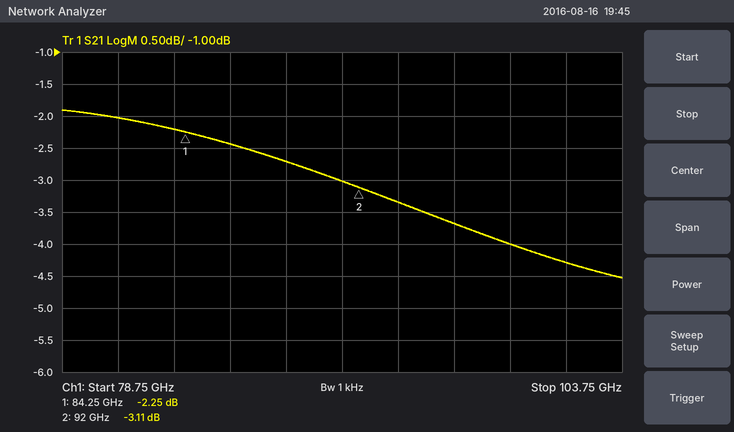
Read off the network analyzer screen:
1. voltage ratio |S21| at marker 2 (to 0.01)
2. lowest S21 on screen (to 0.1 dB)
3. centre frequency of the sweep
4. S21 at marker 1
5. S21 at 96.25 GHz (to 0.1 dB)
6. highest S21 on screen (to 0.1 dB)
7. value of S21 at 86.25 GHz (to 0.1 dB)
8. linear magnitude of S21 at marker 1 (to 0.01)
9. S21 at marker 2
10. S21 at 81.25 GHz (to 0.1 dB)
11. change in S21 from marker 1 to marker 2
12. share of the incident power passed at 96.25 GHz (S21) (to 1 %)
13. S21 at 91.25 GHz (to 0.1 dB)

0.70
-4.5 dB
91.25 GHz
-2.25 dB
-3.7 dB
-1.9 dB
-2.4 dB
0.77
-3.11 dB
-2.0 dB
-0.86 dB
43 %
-3.0 dB
